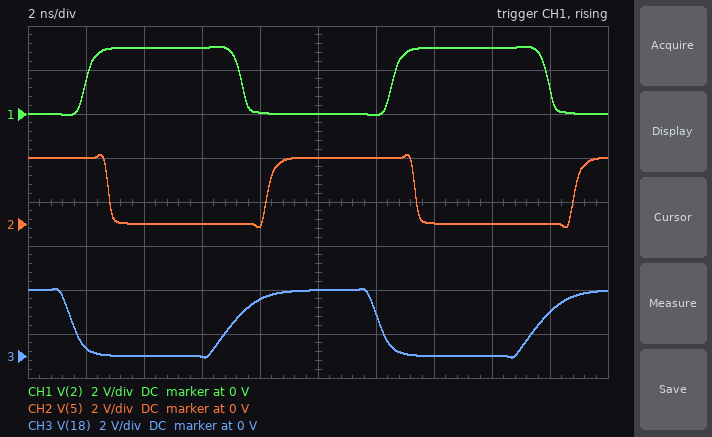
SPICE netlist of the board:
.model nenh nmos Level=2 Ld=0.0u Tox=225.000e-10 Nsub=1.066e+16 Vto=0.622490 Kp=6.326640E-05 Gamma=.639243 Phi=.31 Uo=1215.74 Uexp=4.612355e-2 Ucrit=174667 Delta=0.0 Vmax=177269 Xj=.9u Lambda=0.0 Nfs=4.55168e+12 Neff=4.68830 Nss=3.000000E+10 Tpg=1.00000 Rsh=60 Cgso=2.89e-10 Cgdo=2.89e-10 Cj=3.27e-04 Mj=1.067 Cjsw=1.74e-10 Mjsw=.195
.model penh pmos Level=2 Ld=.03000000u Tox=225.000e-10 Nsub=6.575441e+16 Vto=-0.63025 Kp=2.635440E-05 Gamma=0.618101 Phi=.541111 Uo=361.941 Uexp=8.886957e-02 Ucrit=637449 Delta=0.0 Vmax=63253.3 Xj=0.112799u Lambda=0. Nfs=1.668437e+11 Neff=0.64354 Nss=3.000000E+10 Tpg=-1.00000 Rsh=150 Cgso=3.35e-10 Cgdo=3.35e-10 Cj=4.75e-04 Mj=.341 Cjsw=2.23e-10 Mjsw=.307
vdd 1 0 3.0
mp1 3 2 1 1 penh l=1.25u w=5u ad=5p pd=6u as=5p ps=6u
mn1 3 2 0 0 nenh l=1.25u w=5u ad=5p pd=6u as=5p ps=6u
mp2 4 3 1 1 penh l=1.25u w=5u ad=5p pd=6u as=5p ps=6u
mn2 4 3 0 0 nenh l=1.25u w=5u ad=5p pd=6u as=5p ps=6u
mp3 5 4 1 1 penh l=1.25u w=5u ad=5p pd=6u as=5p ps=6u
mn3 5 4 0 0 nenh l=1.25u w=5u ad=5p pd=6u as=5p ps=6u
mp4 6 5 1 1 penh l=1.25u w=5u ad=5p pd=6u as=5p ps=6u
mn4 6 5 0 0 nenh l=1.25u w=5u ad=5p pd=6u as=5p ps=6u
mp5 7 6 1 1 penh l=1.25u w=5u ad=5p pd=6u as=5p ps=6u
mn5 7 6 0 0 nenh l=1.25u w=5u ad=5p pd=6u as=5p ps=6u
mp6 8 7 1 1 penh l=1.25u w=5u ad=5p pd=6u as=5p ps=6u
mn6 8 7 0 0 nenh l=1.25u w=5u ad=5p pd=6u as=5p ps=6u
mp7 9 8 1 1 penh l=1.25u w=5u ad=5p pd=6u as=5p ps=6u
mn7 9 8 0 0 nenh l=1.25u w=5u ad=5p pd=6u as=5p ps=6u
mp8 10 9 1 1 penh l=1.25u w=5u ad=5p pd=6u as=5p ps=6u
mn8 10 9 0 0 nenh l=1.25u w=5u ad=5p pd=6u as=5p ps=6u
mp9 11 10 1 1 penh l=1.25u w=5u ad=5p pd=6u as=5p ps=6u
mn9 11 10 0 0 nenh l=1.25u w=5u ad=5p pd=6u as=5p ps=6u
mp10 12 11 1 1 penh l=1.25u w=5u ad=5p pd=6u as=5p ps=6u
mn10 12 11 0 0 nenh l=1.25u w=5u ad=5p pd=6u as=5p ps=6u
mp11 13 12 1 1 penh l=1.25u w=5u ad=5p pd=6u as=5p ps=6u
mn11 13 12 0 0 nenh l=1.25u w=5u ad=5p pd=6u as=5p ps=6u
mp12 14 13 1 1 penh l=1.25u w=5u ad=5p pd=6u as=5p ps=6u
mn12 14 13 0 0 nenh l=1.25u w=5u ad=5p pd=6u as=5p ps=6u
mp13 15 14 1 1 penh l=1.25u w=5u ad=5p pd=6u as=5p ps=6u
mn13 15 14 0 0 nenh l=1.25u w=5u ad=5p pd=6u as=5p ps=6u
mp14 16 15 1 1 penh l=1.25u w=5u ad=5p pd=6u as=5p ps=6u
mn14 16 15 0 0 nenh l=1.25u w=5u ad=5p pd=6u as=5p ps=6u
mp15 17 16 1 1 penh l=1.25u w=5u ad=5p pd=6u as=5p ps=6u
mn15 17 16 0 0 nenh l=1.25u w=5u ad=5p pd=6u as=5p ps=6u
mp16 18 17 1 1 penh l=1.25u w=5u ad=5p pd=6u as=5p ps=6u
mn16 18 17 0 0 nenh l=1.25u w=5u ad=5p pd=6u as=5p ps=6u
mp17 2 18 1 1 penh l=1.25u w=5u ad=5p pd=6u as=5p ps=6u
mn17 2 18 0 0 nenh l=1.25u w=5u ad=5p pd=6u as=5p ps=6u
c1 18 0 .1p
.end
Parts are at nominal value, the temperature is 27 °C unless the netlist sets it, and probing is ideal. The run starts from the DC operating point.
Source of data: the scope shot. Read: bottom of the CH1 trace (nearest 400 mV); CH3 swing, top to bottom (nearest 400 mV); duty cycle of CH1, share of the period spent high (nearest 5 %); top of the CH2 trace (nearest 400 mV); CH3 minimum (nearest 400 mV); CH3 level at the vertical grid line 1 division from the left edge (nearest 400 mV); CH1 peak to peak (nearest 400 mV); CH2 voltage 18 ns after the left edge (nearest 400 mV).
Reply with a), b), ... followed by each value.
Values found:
a) 0 V
b) 3.2 V
c) 50 %
d) 3.2 V
e) 0 V
f) 400 mV
g) 3.2 V
h) 0 V
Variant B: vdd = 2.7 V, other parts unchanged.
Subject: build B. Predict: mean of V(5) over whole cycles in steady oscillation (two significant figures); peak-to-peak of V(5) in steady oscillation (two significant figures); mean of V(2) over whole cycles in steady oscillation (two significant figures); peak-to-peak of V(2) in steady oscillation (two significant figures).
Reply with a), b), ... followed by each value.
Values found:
a) 1.3 V
b) 3.0 V
c) 1.4 V
d) 2.8 V
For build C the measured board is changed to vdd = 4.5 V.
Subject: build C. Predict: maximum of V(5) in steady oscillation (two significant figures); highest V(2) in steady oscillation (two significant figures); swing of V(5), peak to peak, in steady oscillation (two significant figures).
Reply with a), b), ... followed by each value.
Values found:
a) 4.7 V
b) 4.6 V
c) 4.9 V
